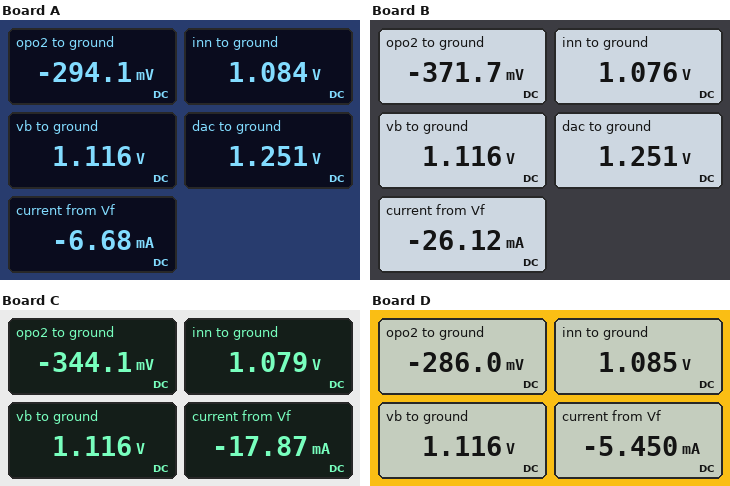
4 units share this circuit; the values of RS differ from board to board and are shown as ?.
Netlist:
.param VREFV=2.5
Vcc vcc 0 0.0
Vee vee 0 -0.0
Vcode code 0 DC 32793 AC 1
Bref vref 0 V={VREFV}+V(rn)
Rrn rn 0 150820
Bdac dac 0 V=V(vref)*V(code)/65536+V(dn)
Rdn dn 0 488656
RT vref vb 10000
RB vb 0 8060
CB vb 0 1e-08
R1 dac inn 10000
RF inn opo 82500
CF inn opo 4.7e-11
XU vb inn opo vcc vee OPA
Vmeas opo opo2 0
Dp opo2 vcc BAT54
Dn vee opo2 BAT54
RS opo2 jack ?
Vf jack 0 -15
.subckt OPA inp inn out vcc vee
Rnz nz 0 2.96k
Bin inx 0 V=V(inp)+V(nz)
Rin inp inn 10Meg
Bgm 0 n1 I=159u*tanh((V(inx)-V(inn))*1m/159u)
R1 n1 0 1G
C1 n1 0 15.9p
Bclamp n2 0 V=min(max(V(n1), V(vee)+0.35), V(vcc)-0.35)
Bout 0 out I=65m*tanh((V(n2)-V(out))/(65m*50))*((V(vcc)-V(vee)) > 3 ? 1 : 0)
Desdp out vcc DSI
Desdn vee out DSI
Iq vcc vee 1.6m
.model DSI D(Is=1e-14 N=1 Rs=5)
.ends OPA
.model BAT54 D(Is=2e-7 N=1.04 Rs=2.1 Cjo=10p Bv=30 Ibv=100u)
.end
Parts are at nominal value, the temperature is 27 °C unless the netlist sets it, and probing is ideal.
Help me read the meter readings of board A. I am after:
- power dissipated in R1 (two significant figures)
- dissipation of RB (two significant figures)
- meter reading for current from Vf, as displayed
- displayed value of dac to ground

2.8 µW
150 µW
-6.68 mA
1.251 V
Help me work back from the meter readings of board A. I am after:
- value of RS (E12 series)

2.2 kΩ
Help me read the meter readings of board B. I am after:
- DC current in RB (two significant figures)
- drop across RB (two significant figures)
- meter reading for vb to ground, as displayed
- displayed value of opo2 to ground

140 µA
1.1 V
1.116 V
-371.7 mV
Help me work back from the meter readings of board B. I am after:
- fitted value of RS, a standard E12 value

560 Ω
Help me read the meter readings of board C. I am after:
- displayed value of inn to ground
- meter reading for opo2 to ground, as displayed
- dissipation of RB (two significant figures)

1.079 V
-344.1 mV
150 µW
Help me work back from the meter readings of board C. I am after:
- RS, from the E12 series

820 Ω
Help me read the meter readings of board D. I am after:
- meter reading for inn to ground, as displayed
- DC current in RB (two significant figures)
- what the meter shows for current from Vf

1.085 V
140 µA
-5.450 mA
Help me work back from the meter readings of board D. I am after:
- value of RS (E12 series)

2.7 kΩ
